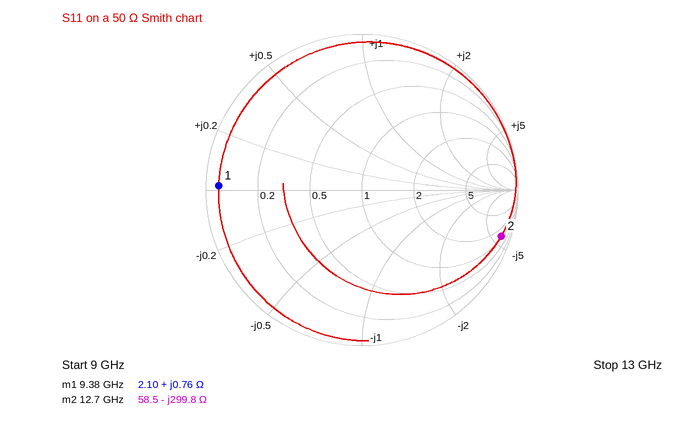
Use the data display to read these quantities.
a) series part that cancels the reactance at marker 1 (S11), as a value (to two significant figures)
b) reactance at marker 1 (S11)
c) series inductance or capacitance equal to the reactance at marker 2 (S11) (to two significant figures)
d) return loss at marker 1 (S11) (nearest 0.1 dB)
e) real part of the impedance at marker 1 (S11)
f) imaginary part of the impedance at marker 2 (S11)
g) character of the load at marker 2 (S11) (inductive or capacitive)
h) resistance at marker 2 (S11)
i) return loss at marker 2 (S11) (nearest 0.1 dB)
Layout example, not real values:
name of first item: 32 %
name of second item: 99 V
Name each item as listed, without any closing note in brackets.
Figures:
series part that cancels the reactance at marker 1 (S11), as a value: 22 pF
reactance at marker 1: +0.76 Ω
series inductance or capacitance equal to the reactance at marker 2 (S11): 42 fF
return loss at marker 1 (S11): 0.7 dB
real part of the impedance at marker 1: 2.10 Ω
imaginary part of the impedance at marker 2: -299.8 Ω
character of the load at marker 2 (S11): capacitive
resistance at marker 2: 58.5 Ω
return loss at marker 2 (S11): 0.5 dB
